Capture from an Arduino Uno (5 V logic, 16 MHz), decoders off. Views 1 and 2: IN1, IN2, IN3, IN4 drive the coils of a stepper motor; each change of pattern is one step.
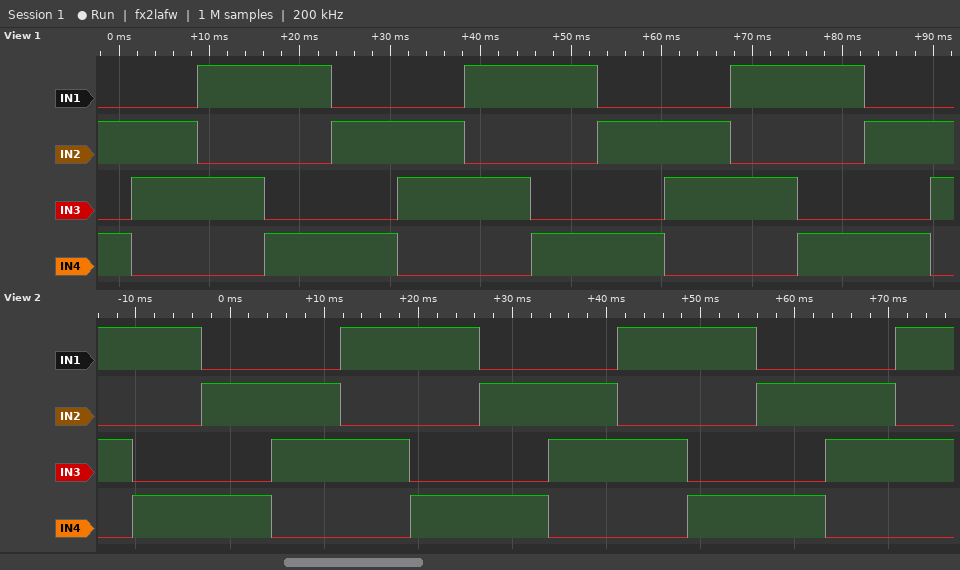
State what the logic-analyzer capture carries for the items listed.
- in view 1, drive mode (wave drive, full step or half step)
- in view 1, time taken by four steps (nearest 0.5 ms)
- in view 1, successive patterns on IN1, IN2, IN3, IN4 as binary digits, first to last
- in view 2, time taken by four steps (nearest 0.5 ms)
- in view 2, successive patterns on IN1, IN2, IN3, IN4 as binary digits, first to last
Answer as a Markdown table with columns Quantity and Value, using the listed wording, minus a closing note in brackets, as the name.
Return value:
| Quantity | Value |
|---|---|
| in view 1, drive mode | full step |
| in view 1, time taken by four steps | 29.5 ms |
| in view 1, successive patterns on IN1, IN2, IN3, IN4 as binary digits, first to last | 0101 0110 1010 1001 0101 0110 1010 1001 0101 0110 1010 1001 0101 0110 |
| in view 2, time taken by four steps | 29.5 ms |
| in view 2, successive patterns on IN1, IN2, IN3, IN4 as binary digits, first to last | 1010 1001 0101 0110 1010 1001 0101 0110 1010 1001 0101 0110 1010 |
